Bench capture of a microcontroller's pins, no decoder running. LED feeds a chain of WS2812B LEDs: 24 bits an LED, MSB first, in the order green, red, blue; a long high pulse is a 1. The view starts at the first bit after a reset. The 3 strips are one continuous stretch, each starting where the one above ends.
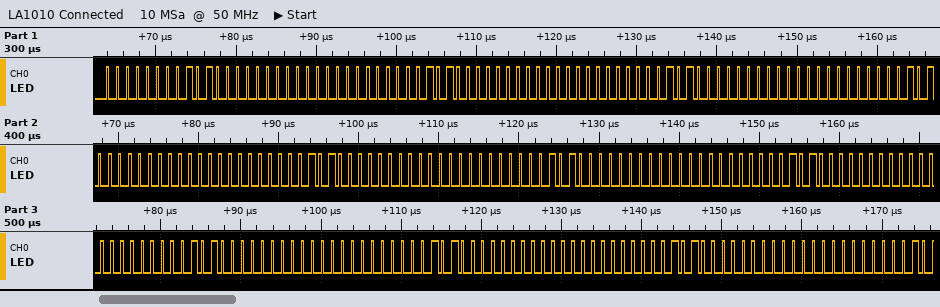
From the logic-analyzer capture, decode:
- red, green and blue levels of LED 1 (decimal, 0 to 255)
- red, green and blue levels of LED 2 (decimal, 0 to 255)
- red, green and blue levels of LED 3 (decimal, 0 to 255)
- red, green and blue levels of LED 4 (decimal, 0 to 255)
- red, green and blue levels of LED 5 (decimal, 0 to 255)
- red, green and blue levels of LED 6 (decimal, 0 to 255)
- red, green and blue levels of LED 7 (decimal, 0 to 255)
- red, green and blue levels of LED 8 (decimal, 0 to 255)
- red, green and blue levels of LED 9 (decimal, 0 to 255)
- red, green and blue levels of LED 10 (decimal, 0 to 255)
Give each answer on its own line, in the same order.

160, 0, 0
160, 0, 0
160, 0, 0
160, 0, 0
160, 0, 0
160, 0, 0
160, 0, 0
160, 0, 0
160, 0, 0
160, 0, 0
